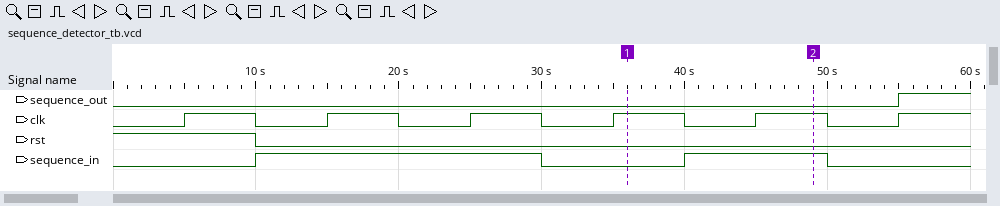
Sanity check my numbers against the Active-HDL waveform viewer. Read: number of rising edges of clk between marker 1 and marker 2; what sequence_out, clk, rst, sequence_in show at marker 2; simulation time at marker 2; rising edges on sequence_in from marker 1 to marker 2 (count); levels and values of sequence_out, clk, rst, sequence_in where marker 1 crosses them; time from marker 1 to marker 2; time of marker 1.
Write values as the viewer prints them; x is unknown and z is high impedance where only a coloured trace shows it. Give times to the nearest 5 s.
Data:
1
sequence_out=0, clk=1, rst=0, sequence_in=1
50 s
1
sequence_out=0, clk=1, rst=0, sequence_in=0
15 s
35 s
